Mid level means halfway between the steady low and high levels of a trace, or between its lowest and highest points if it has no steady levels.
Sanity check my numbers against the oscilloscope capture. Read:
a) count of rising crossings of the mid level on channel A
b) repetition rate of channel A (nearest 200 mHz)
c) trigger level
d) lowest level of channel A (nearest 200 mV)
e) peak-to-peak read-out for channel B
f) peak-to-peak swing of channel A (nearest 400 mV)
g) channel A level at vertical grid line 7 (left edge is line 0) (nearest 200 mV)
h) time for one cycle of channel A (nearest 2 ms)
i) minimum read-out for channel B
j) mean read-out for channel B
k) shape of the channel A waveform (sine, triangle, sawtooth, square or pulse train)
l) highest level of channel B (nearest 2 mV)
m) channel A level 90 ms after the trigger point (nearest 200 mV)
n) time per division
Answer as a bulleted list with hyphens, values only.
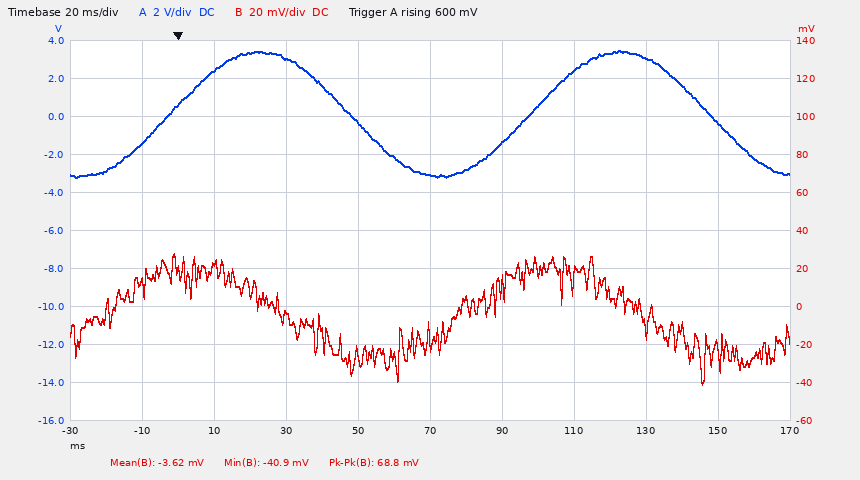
- 2
- 10.0 Hz
- 600 mV
- -3.2 V
- 68.8 mV
- 6.8 V
- 2.4 V
- 100 ms
- -40.9 mV
- -3.62 mV
- sine
- 28 mV
- -1.4 V
- 20 ms
